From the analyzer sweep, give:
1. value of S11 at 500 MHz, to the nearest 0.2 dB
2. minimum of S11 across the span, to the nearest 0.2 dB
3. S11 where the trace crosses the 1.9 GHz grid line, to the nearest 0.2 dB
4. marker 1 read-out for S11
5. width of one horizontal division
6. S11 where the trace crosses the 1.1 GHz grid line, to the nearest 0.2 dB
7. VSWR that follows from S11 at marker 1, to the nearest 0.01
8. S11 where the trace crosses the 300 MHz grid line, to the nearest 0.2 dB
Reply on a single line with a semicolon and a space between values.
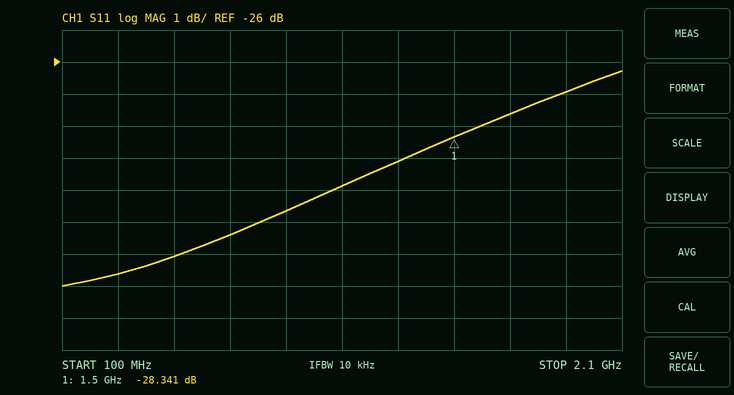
-32.0 dB; -33.0 dB; -27.0 dB; -28.341 dB; 200 MHz; -29.8 dB; 1.08; -32.6 dB
